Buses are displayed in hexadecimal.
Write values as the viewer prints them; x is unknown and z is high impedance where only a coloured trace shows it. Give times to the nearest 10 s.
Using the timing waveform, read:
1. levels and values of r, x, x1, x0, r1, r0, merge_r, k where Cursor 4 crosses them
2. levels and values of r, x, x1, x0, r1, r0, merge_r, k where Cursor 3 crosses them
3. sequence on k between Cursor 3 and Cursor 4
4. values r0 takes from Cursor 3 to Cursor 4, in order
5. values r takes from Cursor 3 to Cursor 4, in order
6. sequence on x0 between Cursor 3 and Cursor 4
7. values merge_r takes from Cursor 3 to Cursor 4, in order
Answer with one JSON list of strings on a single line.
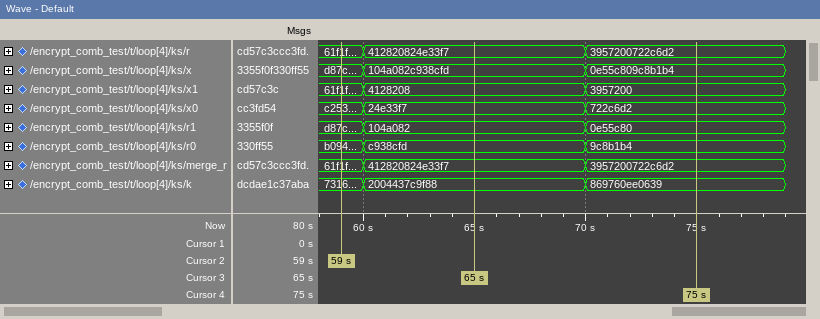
["r=3957200722c6d2, x=0e55c809c8b1b4, x1=3957200, x0=722c6d2, r1=0e55c80, r0=9c8b1b4, merge_r=3957200722c6d2, k=869760ee0639", "r=412820824e33f7, x=104a082c938cfd, x1=4128208, x0=24e33f7, r1=104a082, r0=c938cfd, merge_r=412820824e33f7, k=2004437c9f88", "2004437c9f88, 869760ee0639", "c938cfd, 9c8b1b4", "412820824e33f7, 3957200722c6d2", "24e33f7, 722c6d2", "412820824e33f7, 3957200722c6d2"]
